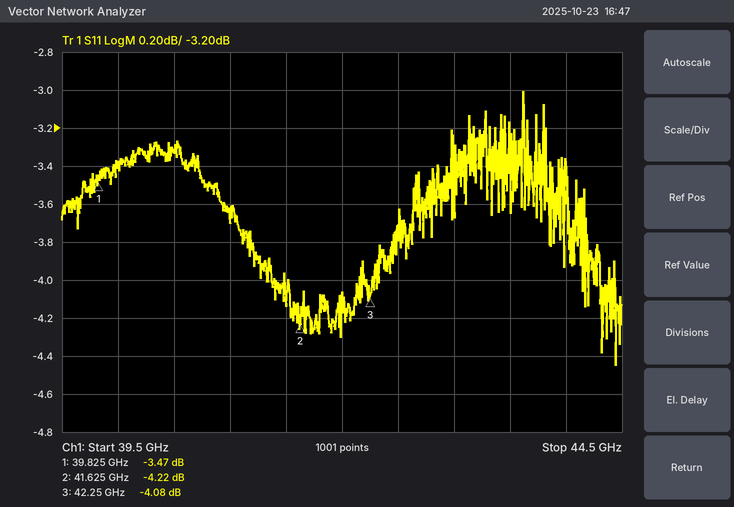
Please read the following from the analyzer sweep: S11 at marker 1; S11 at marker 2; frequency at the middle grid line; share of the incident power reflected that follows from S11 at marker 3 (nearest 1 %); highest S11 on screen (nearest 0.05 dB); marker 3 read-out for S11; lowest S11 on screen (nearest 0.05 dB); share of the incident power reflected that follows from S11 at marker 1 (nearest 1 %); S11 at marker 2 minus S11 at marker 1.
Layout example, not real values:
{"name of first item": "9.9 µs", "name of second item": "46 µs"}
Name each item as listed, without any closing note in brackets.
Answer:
{"S11 at marker 1": "-3.47 dB", "S11 at marker 2": "-4.22 dB", "frequency at the middle grid line": "42 GHz", "share of the incident power reflected that follows from S11 at marker 3": "39 %", "highest S11 on screen": "-3.00 dB", "marker 3 read-out for S11": "-4.08 dB", "lowest S11 on screen": "-4.45 dB", "share of the incident power reflected that follows from S11 at marker 1": "45 %", "S11 at marker 2 minus S11 at marker 1": "-0.75 dB"}
